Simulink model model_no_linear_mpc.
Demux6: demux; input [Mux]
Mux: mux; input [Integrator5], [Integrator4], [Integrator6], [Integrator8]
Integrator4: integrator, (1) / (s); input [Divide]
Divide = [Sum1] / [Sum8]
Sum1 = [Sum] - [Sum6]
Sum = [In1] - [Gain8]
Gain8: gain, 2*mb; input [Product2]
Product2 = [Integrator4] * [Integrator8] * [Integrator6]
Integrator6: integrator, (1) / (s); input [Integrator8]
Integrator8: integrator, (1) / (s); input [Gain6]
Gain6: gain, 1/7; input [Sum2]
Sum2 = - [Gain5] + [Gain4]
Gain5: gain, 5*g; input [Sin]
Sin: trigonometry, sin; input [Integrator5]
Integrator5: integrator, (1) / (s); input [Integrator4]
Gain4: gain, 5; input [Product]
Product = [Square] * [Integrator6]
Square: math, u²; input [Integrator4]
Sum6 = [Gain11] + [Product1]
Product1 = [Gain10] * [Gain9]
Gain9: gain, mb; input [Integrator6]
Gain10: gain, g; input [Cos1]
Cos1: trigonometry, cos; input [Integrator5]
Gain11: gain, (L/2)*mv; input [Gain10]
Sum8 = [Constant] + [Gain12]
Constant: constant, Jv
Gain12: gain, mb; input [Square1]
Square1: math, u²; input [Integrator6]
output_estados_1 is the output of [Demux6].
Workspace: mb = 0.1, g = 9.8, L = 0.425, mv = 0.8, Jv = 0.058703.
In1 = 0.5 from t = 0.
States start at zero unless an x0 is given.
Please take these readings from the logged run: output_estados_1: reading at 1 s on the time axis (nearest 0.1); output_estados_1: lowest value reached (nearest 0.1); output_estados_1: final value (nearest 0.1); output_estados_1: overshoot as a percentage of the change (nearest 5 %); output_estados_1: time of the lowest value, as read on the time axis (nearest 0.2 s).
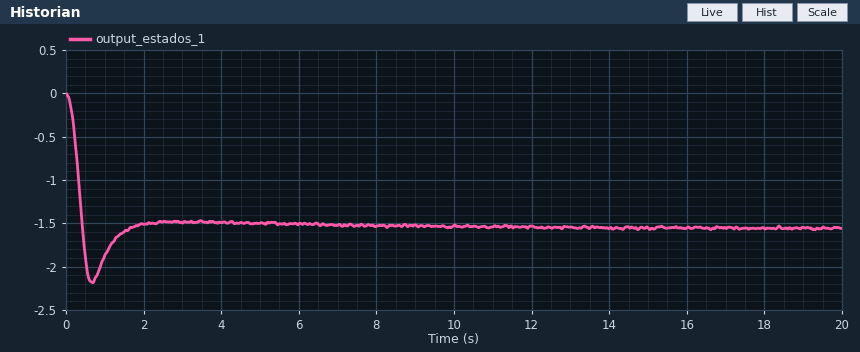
-1.9
-2.2
-1.6
40 %
0.6 s
